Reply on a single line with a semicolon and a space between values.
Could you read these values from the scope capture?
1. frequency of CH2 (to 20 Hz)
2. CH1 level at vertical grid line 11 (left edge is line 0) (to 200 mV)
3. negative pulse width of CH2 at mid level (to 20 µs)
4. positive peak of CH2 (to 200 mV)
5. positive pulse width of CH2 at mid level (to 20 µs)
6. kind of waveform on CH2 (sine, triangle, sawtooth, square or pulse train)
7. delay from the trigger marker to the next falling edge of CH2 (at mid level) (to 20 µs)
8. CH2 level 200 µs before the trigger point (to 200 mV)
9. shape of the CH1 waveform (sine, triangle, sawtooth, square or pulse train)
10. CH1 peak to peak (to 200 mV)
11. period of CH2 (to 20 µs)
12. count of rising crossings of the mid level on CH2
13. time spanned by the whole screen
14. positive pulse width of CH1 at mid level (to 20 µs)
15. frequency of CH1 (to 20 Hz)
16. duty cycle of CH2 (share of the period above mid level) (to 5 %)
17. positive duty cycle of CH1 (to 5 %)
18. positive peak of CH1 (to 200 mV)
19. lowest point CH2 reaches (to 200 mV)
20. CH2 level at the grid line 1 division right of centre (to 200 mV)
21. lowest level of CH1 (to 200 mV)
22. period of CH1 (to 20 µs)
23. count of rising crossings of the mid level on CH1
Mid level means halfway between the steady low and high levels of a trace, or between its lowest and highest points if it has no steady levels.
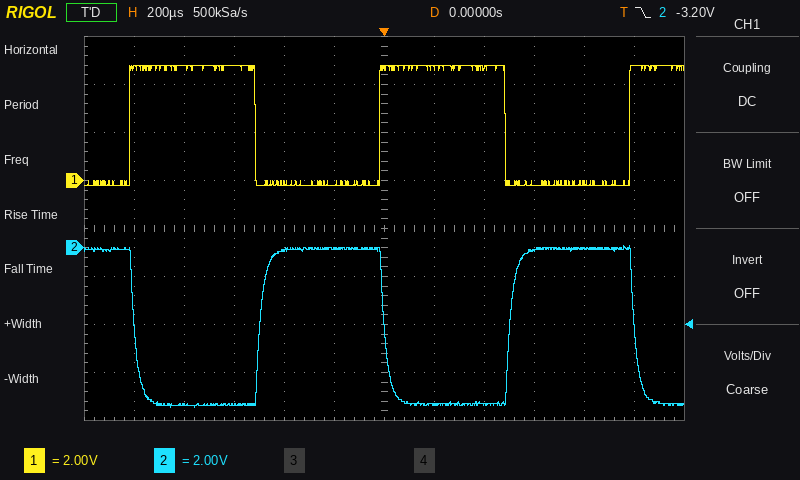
1.00 kHz; 4.8 V; 500 µs; 0.0 V; 500 µs; square; 1.00 ms; 0.0 V; square; 5.0 V; 1.00 ms; 2; 2.4 ms; 500 µs; 1.00 kHz; 50 %; 50 %; 4.8 V; -6.6 V; -6.6 V; -200 mV; 1.00 ms; 3
